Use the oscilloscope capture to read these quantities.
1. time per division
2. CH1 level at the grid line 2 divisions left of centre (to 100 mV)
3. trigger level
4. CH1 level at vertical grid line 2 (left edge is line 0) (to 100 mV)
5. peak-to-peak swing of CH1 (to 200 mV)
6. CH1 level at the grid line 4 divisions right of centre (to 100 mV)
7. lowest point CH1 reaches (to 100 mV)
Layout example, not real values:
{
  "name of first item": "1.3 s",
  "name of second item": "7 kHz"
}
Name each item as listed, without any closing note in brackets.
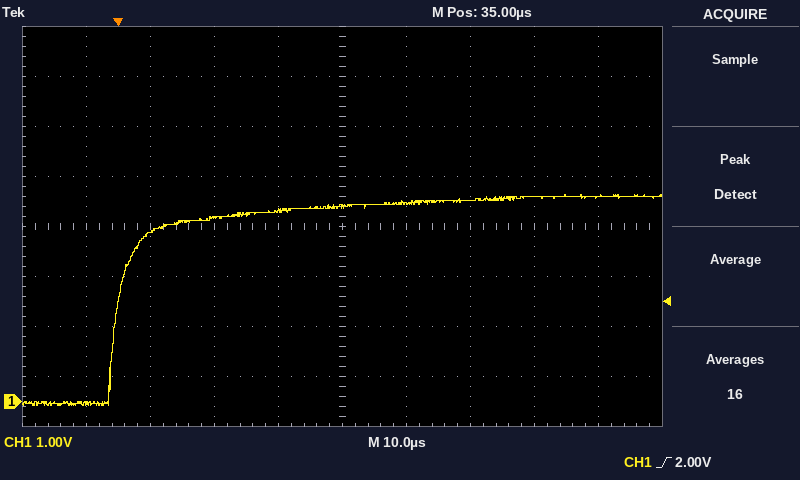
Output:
{
  "time per division": "10 µs",
  "CH1 level at the grid line 2 divisions left of centre": "3.7 V",
  "trigger level": "2.00 V",
  "CH1 level at vertical grid line 2 (left edge is line 0)": "3.4 V",
  "peak-to-peak swing of CH1": "4.2 V",
  "CH1 level at the grid line 4 divisions right of centre": "4.1 V",
  "lowest point CH1 reaches": "-100 mV"
}
